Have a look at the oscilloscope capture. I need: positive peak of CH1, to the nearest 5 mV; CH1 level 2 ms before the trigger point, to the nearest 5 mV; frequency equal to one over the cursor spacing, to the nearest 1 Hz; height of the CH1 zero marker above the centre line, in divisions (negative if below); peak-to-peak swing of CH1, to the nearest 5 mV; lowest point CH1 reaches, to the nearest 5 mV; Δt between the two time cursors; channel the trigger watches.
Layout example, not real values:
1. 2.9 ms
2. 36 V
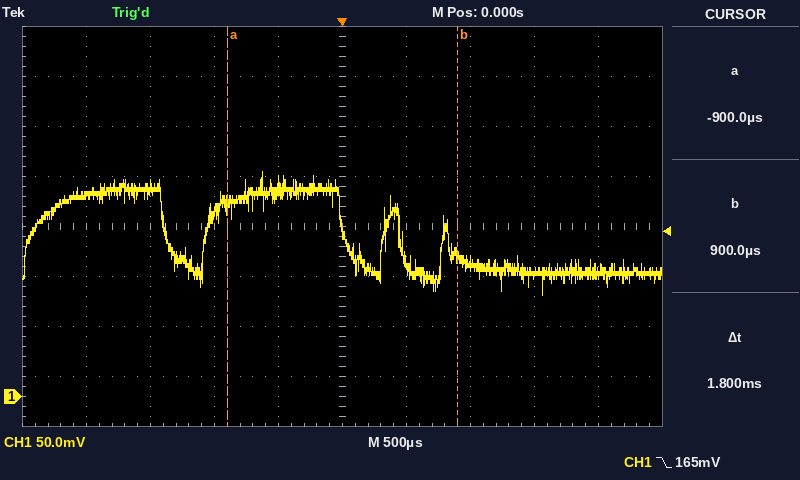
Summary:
1. 225 mV
2. 200 mV
3. 556 Hz
4. -3.4 div
5. 125 mV
6. 100 mV
7. 1.8 ms
8. CH1
